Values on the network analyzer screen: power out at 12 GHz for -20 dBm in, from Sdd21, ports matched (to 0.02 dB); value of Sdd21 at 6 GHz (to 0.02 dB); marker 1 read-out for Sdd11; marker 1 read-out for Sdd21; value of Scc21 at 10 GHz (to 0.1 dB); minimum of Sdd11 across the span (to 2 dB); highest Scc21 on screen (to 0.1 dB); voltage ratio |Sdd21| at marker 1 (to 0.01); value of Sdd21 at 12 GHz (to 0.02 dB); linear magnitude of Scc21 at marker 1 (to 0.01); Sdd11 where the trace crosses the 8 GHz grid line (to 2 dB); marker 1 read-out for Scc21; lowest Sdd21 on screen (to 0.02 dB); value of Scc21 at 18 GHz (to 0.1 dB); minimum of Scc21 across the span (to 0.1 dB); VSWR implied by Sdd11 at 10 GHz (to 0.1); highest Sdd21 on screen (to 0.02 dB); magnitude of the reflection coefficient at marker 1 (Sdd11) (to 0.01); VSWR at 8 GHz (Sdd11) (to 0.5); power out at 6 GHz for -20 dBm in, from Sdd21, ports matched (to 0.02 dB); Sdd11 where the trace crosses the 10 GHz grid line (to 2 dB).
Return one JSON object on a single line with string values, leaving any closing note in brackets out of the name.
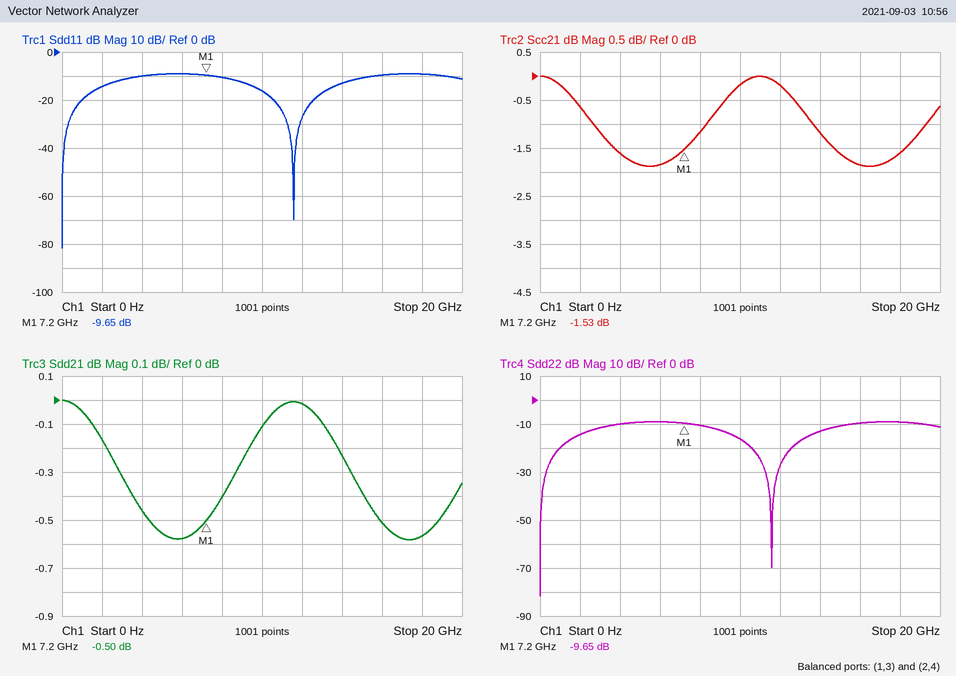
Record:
{"power out at 12 GHz for -20 dBm in, from Sdd21, ports matched": "-20.02 dBm", "value of Sdd21 at 6 GHz": "-0.58 dB", "marker 1 read-out for Sdd11": "-9.65 dB", "marker 1 read-out for Sdd21": "-0.50 dB", "value of Scc21 at 10 GHz": "-0.2 dB", "minimum of Sdd11 across the span": "-82 dB", "highest Scc21 on screen": "0.0 dB", "voltage ratio |Sdd21| at marker 1": "0.94", "value of Sdd21 at 12 GHz": "-0.02 dB", "linear magnitude of Scc21 at marker 1": "0.84", "Sdd11 where the trace crosses the 8 GHz grid line": "-10 dB", "marker 1 read-out for Scc21": "-1.53 dB", "lowest Sdd21 on screen": "-0.58 dB", "value of Scc21 at 18 GHz": "-1.6 dB", "minimum of Scc21 across the span": "-1.9 dB", "VSWR implied by Sdd11 at 10 GHz": "1.4", "highest Sdd21 on screen": "0.00 dB", "magnitude of the reflection coefficient at marker 1 (Sdd11)": "0.33", "VSWR at 8 GHz (Sdd11)": "2.0", "power out at 6 GHz for -20 dBm in, from Sdd21, ports matched": "-20.58 dBm", "Sdd11 where the trace crosses the 10 GHz grid line": "-16 dB"}
